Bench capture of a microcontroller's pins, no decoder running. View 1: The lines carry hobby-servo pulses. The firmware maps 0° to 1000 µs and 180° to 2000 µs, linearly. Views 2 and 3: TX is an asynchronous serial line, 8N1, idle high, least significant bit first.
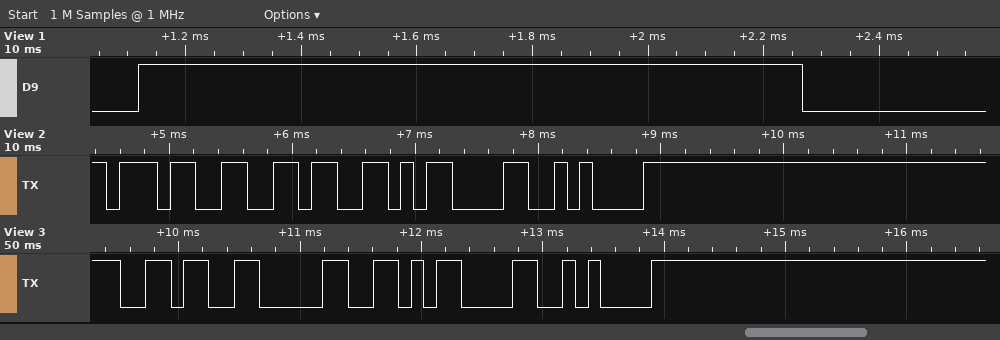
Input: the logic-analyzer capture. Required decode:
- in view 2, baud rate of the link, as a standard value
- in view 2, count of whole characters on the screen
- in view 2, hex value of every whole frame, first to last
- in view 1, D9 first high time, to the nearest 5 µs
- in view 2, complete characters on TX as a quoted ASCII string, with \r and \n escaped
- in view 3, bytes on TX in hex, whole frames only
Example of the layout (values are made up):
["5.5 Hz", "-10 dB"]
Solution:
["9600 baud", "4", "37 36 0D 0A", "1150 µs", "\"76\\r\\n\"", "36 30 0D 0A"]
